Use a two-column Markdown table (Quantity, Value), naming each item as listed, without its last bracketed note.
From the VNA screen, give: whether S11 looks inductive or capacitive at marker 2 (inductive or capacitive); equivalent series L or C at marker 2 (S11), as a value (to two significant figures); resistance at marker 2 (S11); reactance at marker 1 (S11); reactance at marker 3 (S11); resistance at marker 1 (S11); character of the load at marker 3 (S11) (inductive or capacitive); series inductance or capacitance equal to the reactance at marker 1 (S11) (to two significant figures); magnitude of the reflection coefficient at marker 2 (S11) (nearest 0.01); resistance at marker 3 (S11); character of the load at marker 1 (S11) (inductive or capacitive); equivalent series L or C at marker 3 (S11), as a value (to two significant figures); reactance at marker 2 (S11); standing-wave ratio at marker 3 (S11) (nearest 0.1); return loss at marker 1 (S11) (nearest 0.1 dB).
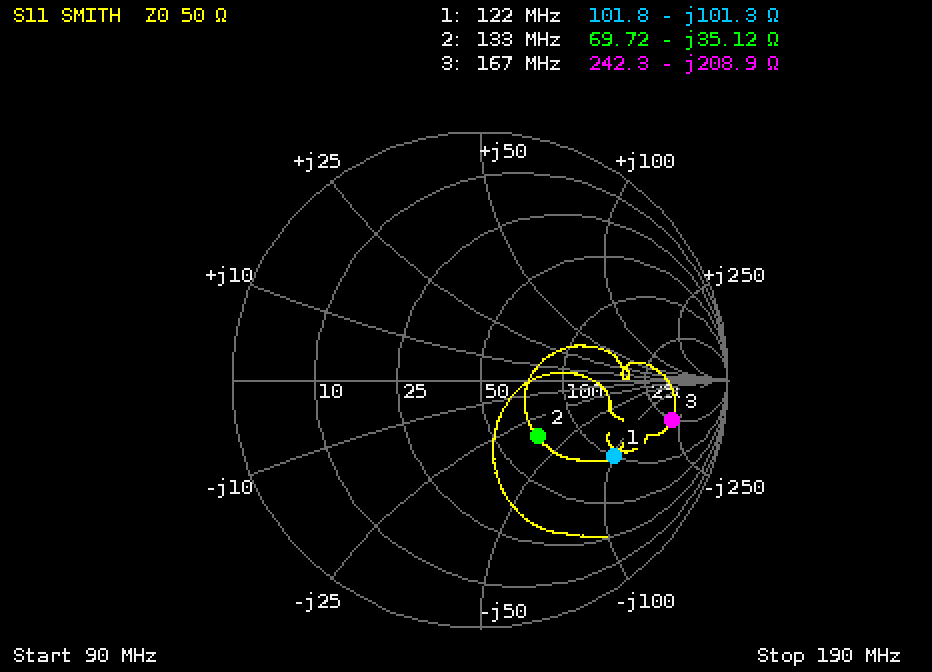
| Quantity | Value |
|---|---|
| whether S11 looks inductive or capacitive at marker 2 | capacitive |
| equivalent series L or C at marker 2 (S11), as a value | 34 pF |
| resistance at marker 2 | 69.72 Ω |
| reactance at marker 1 | -101.3 Ω |
| reactance at marker 3 | -208.9 Ω |
| resistance at marker 1 | 101.8 Ω |
| character of the load at marker 3 (S11) | capacitive |
| series inductance or capacitance equal to the reactance at marker 1 (S11) | 13 pF |
| magnitude of the reflection coefficient at marker 2 (S11) | 0.32 |
| resistance at marker 3 | 242.3 Ω |
| character of the load at marker 1 (S11) | capacitive |
| equivalent series L or C at marker 3 (S11), as a value | 4.6 pF |
| reactance at marker 2 | -35.12 Ω |
| standing-wave ratio at marker 3 (S11) | 8.5 |
| return loss at marker 1 (S11) | 4.1 dB |
